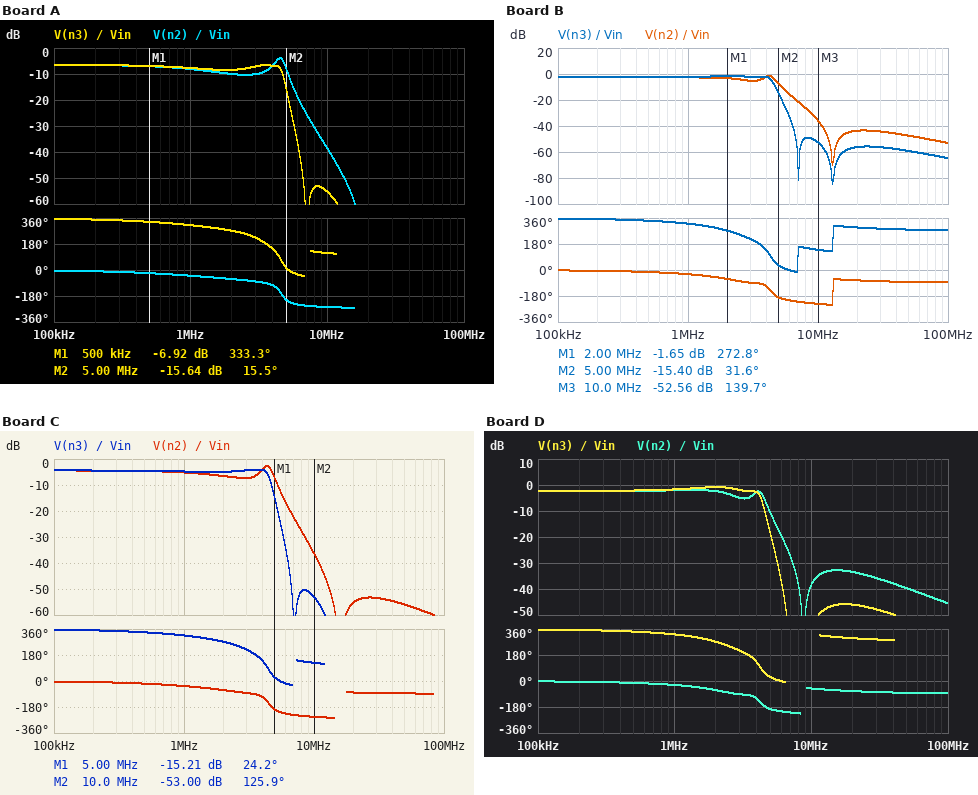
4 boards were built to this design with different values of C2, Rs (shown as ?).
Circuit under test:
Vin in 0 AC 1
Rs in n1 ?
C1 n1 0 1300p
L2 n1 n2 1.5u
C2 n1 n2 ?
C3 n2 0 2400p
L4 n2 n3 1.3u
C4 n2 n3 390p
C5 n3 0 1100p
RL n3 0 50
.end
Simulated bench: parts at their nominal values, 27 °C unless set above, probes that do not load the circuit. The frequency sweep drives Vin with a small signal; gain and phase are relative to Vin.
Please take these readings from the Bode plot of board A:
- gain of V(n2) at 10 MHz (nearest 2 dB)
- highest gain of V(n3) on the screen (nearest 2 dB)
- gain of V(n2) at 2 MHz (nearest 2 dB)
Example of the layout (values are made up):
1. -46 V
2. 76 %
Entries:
1. -38 dB
2. -6 dB
3. -10 dB
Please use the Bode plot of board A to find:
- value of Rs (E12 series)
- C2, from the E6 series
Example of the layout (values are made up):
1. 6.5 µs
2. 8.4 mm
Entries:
1. 56 Ω
2. 47 pF
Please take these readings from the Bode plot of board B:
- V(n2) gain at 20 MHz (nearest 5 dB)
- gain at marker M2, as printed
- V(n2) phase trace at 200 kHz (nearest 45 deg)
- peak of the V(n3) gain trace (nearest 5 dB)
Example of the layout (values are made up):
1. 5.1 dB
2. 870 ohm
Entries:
1. -45 dB
2. -15.40 dB
3. 0 deg
4. 0 dB
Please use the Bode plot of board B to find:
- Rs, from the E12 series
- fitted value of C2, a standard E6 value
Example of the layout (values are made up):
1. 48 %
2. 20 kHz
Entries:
1. 18 Ω
2. 100 pF
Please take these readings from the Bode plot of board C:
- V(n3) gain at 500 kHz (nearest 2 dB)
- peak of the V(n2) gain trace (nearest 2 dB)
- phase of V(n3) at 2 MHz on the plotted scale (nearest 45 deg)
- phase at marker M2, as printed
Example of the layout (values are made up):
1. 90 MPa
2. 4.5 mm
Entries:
1. -4 dB
2. -2 dB
3. 270 deg
4. 125.9 deg
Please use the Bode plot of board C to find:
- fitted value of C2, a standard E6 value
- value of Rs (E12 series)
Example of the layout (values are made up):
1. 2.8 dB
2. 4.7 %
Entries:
1. 68 pF
2. 33 Ω
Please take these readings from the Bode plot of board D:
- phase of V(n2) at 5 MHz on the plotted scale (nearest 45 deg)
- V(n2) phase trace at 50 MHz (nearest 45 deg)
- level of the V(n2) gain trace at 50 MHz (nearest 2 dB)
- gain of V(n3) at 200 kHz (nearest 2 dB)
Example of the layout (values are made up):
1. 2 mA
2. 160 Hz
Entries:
1. -180 deg
2. -90 deg
3. -40 dB
4. -2 dB
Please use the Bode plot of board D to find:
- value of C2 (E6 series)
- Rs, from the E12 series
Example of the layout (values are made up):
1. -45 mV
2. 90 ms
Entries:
1. 220 pF
2. 15 Ω
